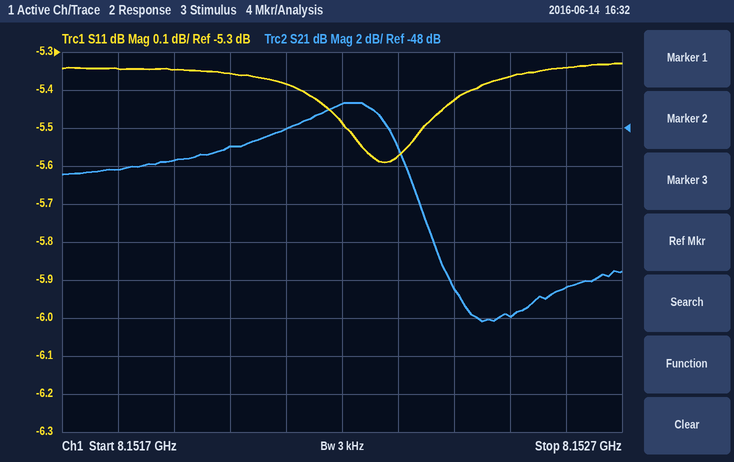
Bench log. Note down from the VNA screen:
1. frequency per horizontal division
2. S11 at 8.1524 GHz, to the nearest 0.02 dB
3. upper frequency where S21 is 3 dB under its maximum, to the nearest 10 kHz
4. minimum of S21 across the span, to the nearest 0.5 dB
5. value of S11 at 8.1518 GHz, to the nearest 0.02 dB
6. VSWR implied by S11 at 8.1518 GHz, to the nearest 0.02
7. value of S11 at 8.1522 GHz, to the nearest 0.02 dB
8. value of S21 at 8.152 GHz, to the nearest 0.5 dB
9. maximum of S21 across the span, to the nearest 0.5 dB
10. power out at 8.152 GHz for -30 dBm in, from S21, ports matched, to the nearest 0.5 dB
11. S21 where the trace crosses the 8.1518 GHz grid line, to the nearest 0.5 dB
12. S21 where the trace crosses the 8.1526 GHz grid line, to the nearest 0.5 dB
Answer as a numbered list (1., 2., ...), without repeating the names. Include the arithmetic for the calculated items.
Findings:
1. 100 kHz
2. -5.42 dB
3. 8.15231 GHz
4. -58.0 dB
5. -5.34 dB
6. |Γ| = 10^(-5.34/20) = 0.5408; VSWR = (1 + 0.5408)/(1 − 0.5408) ≈ 3.35, so 3.36 to the nearest 0.02
7. -5.48 dB
8. -49.0 dB
9. -46.5 dB
10. -30 dBm + (-49.0 dB) = -79.0 dBm
11. -50.0 dB
12. -56.5 dB
